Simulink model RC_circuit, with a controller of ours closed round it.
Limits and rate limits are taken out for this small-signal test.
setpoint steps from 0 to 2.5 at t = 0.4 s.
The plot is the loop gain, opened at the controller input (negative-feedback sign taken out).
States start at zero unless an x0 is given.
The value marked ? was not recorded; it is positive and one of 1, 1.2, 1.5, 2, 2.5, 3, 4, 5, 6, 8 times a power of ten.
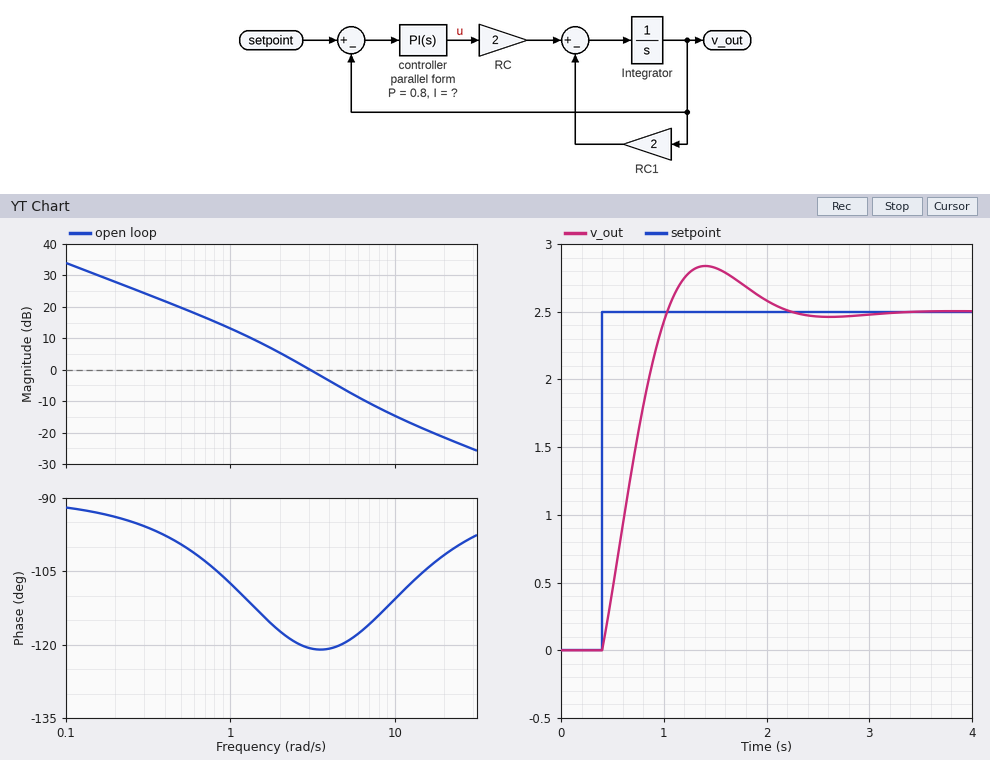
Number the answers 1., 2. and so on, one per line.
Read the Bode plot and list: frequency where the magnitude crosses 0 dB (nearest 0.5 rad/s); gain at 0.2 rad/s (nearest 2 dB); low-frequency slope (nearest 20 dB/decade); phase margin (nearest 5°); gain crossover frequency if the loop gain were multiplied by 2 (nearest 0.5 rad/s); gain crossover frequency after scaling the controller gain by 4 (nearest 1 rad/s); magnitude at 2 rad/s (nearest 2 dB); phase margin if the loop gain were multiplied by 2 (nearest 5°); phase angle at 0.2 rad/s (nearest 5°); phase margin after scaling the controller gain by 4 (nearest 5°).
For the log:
1. 3.0 rad/s
2. 28 dB
3. -20 dB/decade
4. 60°
5. 5.0 rad/s
6. 8 rad/s
7. 6 dB
8. 60°
9. -95°
10. 65°
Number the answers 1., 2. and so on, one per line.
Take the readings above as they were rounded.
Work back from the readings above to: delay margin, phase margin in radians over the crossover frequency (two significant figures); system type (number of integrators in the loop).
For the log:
1. 0.35 s
2. 1
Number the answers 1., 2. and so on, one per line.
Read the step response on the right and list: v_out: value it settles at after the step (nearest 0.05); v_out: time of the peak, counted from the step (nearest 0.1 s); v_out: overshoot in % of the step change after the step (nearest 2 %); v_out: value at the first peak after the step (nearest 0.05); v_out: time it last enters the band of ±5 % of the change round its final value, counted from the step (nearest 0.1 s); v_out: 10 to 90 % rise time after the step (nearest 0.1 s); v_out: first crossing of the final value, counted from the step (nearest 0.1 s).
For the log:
1. 2.50
2. 1.0 s
3. 14 %
4. 2.85
5. 1.5 s
6. 0.5 s
7. 0.6 s
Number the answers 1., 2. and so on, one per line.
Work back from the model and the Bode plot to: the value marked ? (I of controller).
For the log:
1. 5
